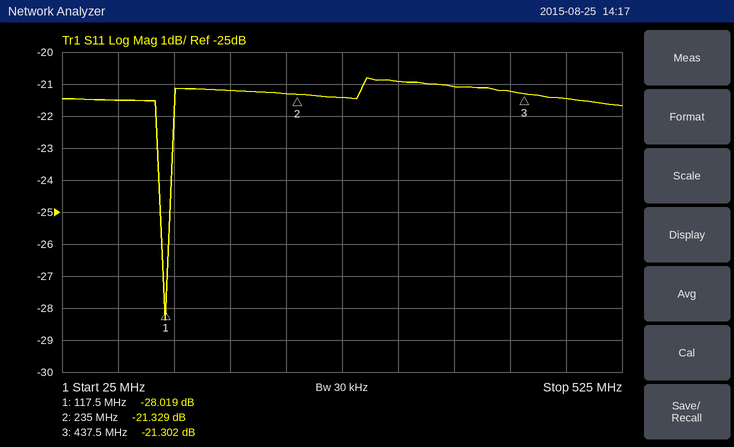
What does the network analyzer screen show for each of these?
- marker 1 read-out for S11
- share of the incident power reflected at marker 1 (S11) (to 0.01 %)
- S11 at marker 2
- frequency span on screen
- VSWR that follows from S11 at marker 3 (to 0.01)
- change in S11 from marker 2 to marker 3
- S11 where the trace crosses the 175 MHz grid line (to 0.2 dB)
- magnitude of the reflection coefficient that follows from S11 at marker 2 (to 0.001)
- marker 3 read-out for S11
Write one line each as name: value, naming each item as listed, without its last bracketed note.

marker 1 read-out for S11: -28.019 dB
share of the incident power reflected at marker 1 (S11): 0.16 %
S11 at marker 2: -21.329 dB
frequency span on screen: 500 MHz
VSWR that follows from S11 at marker 3: 1.19
change in S11 from marker 2 to marker 3: 0.027 dB
S11 where the trace crosses the 175 MHz grid line: -21.2 dB
magnitude of the reflection coefficient that follows from S11 at marker 2: 0.086
marker 3 read-out for S11: -21.302 dB
